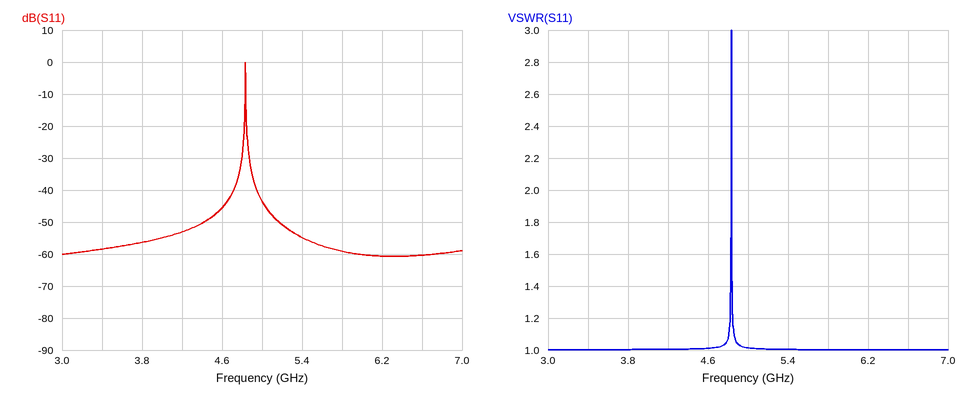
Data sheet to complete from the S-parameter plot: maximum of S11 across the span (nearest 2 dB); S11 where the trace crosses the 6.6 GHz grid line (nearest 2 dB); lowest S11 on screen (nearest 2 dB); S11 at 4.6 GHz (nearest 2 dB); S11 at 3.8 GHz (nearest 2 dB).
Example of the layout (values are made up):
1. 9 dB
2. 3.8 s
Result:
1. 0 dB
2. -60 dB
3. -60 dB
4. -46 dB
5. -56 dB
